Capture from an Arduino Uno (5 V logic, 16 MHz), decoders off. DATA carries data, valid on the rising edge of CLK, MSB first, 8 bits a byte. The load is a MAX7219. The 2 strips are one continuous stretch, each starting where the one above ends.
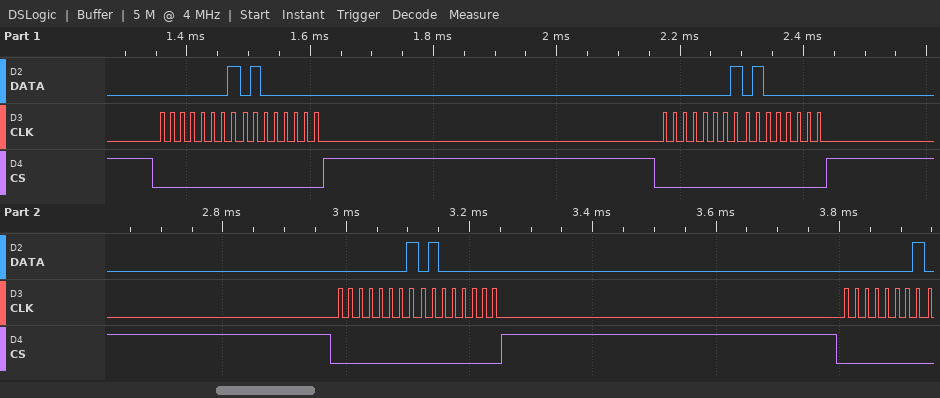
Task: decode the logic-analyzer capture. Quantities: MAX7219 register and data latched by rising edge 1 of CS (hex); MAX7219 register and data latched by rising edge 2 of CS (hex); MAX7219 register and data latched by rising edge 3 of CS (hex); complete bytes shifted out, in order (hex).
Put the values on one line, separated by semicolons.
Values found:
register 0x1, data 0x40; register 0x1, data 0x40; register 0x1, data 0x40; 0x01 0x40 0x01 0x40 0x01 0x40 0x01
